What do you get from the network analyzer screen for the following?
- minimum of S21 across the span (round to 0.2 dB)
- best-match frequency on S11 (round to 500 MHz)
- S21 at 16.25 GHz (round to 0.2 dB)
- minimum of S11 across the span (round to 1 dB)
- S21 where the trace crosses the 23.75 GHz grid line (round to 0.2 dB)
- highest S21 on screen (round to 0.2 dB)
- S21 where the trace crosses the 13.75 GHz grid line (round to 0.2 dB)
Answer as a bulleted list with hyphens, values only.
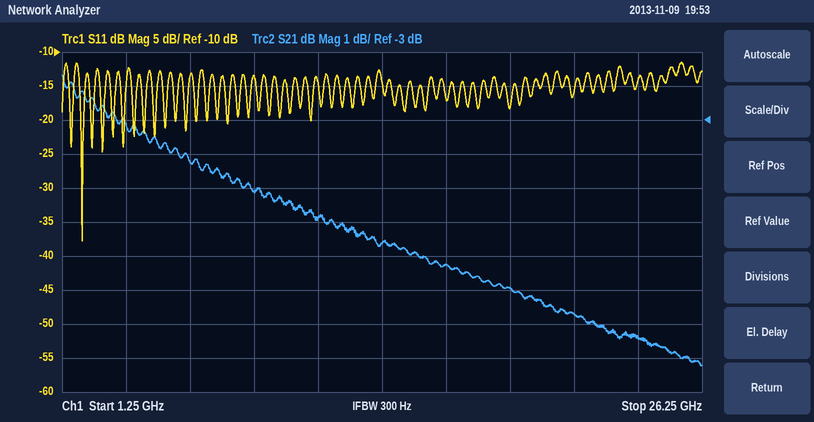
- -10.2 dB
- 2.0 GHz
- -7.2 dB
- -38 dB
- -9.4 dB
- -1.6 dB
- -6.6 dB
